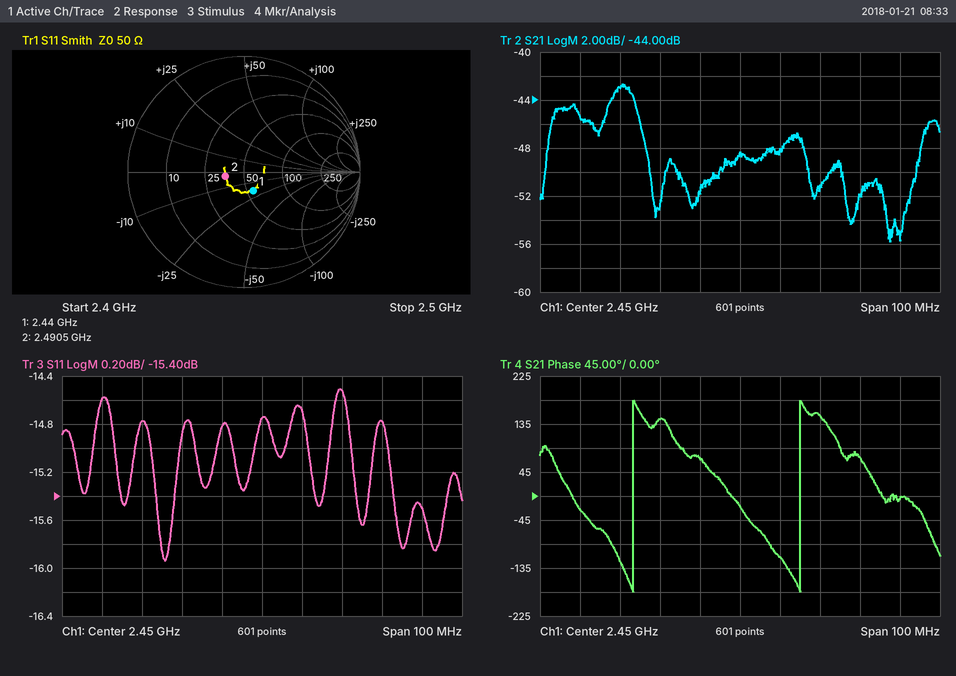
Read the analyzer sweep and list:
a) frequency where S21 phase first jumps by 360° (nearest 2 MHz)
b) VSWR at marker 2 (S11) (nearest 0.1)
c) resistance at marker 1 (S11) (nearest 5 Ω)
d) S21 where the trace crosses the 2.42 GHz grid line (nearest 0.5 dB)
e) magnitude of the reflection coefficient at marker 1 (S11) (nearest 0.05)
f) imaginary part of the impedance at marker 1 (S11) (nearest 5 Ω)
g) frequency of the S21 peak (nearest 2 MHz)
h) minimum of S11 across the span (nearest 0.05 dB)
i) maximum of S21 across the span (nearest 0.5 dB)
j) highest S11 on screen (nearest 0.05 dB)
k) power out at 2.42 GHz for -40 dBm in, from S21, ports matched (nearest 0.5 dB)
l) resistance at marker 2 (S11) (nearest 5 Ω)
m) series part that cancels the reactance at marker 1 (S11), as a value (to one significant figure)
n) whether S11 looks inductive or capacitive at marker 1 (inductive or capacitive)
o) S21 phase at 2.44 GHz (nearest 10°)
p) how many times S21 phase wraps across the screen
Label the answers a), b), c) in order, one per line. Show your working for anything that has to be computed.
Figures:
a) 2.424 GHz
b) 1.4
c) 55 Ω
d) -43.0 dB
e) 0.20
f) -20 Ω
g) 2.420 GHz
h) -15.95 dB
i) -42.5 dB
j) -14.50 dB
k) -40 dBm + (-43.0 dB) = -83.0 dBm
l) 35 Ω
m) L = 20 Ω/(2π × 2.44 GHz) ≈ 1 nH
n) capacitive
o) 70°
p) 2
